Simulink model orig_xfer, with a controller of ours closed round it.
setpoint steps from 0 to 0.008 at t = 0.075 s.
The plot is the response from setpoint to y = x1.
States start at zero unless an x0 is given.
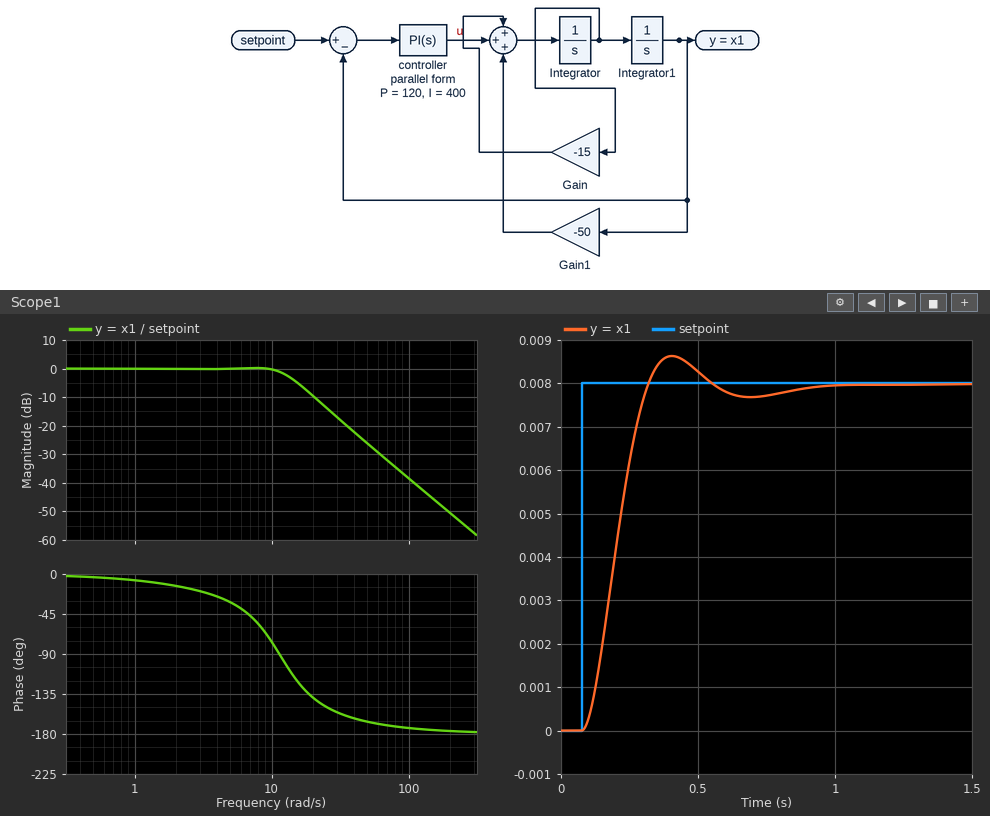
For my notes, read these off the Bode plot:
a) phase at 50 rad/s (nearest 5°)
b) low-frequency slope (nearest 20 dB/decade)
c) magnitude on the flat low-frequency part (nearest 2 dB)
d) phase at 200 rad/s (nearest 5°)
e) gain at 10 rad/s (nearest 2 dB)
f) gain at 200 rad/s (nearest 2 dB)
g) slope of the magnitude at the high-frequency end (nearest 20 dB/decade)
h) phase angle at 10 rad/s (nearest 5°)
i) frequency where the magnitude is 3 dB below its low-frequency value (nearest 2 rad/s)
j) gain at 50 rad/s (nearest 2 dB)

-165°
0 dB/decade
0 dB
-175°
0 dB
-50 dB
-40 dB/decade
-75°
14 rad/s
-26 dB
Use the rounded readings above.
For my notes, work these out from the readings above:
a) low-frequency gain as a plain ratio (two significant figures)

1.0
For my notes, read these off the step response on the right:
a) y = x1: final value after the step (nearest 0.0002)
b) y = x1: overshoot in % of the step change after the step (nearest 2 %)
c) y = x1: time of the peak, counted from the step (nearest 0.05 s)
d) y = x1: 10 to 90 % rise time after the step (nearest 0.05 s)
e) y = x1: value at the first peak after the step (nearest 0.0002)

0.0080
8 %
0.35 s
0.15 s
0.0086
